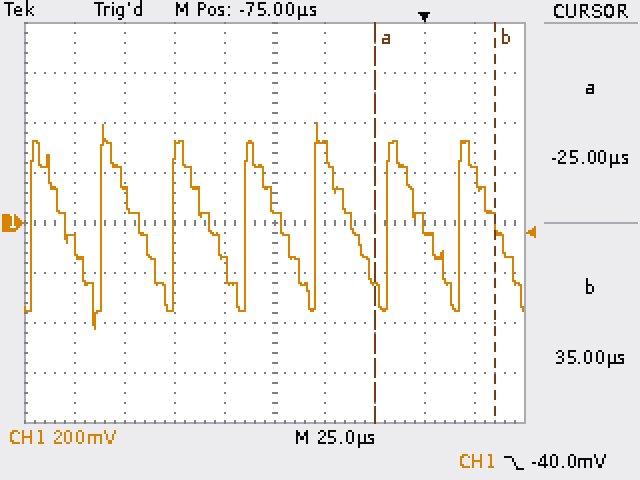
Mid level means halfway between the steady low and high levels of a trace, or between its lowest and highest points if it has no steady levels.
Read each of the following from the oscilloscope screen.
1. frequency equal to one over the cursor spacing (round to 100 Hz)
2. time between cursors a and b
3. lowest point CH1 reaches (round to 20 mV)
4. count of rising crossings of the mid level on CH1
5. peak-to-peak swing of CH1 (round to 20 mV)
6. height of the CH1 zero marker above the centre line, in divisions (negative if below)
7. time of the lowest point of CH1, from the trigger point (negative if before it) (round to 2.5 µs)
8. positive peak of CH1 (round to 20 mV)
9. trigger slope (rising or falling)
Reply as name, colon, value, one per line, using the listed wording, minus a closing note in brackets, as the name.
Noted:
frequency equal to one over the cursor spacing: 16.7 kHz
time between cursors a and b: 60.0 µs
lowest point CH1 reaches: -420 mV
count of rising crossings of the mid level on CH1: 7
peak-to-peak swing of CH1: 820 mV
height of the CH1 zero marker above the centre line, in divisions: 0.0 div
time of the lowest point of CH1, from the trigger point (negative if before it): -165.0 µs
positive peak of CH1: 400 mV
trigger slope: falling
